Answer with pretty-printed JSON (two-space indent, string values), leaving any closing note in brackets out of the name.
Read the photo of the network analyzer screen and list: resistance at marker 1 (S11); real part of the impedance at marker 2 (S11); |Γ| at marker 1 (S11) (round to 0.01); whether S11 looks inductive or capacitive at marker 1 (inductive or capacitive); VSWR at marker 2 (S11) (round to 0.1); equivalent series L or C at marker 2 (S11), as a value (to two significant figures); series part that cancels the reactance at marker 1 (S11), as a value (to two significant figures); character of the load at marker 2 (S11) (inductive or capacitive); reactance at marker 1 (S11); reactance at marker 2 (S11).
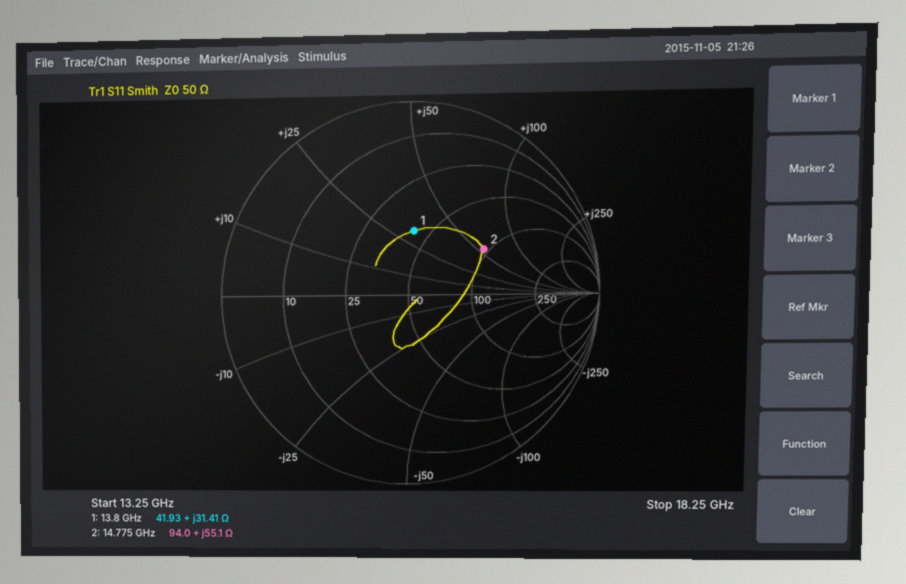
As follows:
{
  "resistance at marker 1": "41.93 Ω",
  "real part of the impedance at marker 2": "94.0 Ω",
  "|Γ| at marker 1 (S11)": "0.33",
  "whether S11 looks inductive or capacitive at marker 1": "inductive",
  "VSWR at marker 2 (S11)": "2.7",
  "equivalent series L or C at marker 2 (S11), as a value": "590 pH",
  "series part that cancels the reactance at marker 1 (S11), as a value": "370 fF",
  "character of the load at marker 2 (S11)": "inductive",
  "reactance at marker 1": "+31.41 Ω",
  "reactance at marker 2": "+55.1 Ω"
}
